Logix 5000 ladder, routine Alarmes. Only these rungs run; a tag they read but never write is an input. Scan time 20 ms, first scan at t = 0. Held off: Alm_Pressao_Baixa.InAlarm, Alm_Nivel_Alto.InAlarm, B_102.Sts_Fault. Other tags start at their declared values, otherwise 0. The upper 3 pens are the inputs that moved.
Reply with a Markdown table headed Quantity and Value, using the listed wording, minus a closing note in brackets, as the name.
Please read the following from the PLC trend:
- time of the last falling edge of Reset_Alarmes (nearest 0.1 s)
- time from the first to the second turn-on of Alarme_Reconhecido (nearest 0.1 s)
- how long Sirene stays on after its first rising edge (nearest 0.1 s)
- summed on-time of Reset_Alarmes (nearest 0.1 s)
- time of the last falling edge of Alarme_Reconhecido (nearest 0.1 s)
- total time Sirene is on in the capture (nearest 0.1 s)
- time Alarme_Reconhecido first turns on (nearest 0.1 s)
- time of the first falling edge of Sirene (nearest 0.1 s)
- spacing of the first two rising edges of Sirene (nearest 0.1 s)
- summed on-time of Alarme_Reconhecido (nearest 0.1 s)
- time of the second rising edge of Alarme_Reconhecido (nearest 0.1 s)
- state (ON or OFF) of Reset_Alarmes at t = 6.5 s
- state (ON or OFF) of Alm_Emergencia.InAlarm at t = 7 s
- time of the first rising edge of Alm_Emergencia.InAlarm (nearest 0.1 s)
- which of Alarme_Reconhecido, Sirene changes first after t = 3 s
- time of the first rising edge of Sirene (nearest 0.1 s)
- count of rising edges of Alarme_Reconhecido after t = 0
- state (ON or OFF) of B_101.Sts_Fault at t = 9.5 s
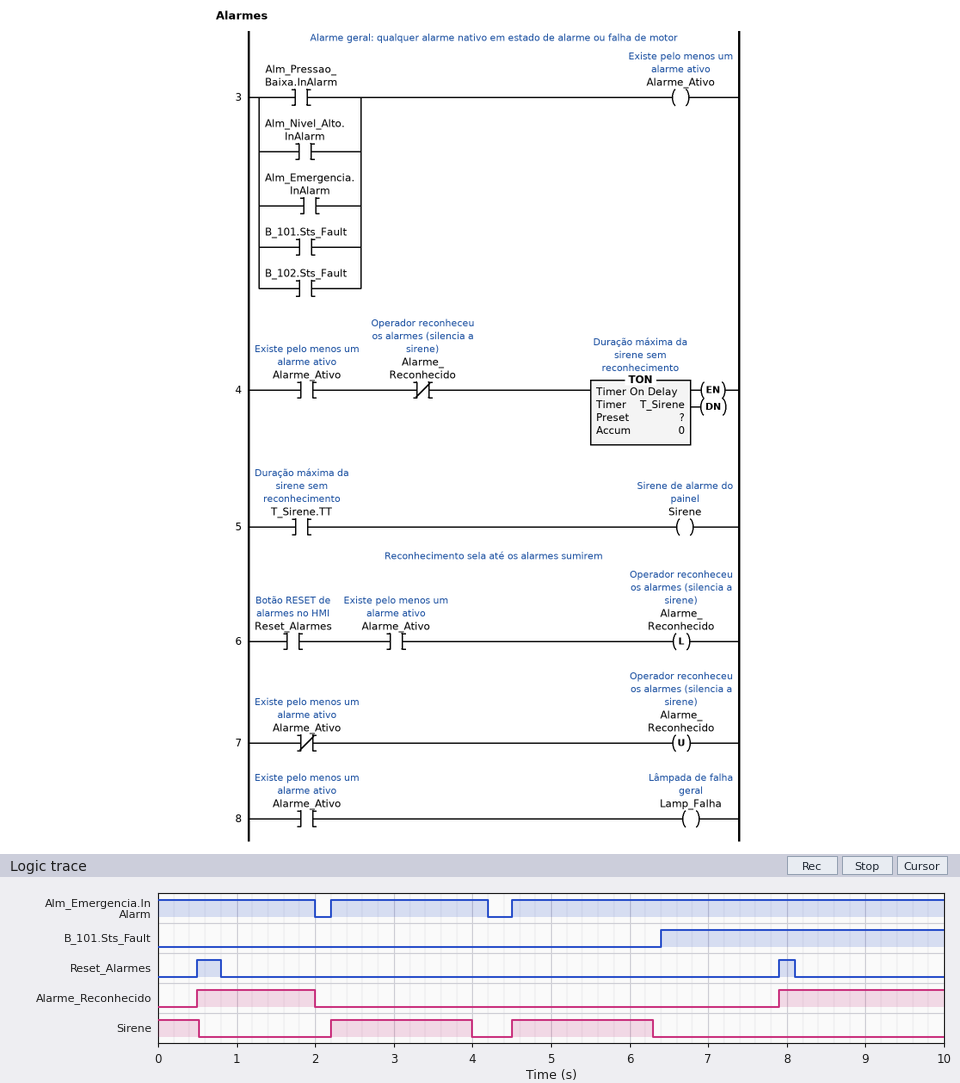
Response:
| Quantity | Value |
|---|---|
| time of the last falling edge of Reset_Alarmes | 8.1 s |
| time from the first to the second turn-on of Alarme_Reconhecido | 7.4 s |
| how long Sirene stays on after its first rising edge | 1.8 s |
| summed on-time of Reset_Alarmes | 0.5 s |
| time of the last falling edge of Alarme_Reconhecido | 2.0 s |
| total time Sirene is on in the capture | 4.1 s |
| time Alarme_Reconhecido first turns on | 0.5 s |
| time of the first falling edge of Sirene | 0.5 s |
| spacing of the first two rising edges of Sirene | 2.3 s |
| summed on-time of Alarme_Reconhecido | 3.6 s |
| time of the second rising edge of Alarme_Reconhecido | 7.9 s |
| state (ON or OFF) of Reset_Alarmes at t = 6.5 s | OFF |
| state (ON or OFF) of Alm_Emergencia.InAlarm at t = 7 s | ON |
| time of the first rising edge of Alm_Emergencia.InAlarm | 2.2 s |
| which of Alarme_Reconhecido, Sirene changes first after t = 3 s | Sirene |
| time of the first rising edge of Sirene | 2.2 s |
| count of rising edges of Alarme_Reconhecido after t = 0 | 2 |
| state (ON or OFF) of B_101.Sts_Fault at t = 9.5 s | ON |
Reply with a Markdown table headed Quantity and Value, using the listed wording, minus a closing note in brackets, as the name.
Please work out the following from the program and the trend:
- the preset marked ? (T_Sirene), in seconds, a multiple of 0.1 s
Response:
| Quantity | Value |
|---|---|
| the preset marked ? (T_Sirene), in seconds, a multiple of 0.1 s | 1.8 s |
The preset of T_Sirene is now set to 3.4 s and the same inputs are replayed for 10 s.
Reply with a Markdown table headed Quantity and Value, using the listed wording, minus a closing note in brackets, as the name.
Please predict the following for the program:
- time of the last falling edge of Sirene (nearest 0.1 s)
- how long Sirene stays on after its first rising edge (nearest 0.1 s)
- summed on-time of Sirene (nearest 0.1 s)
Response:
| Quantity | Value |
|---|---|
| time of the last falling edge of Sirene | 7.9 s |
| how long Sirene stays on after its first rising edge | 2.0 s |
| summed on-time of Sirene | 5.9 s |
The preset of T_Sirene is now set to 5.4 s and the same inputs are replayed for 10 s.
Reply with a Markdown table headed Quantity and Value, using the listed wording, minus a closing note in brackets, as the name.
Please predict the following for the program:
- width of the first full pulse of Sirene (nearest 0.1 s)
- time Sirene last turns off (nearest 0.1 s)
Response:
| Quantity | Value |
|---|---|
| width of the first full pulse of Sirene | 2.0 s |
| time Sirene last turns off | 7.9 s |
